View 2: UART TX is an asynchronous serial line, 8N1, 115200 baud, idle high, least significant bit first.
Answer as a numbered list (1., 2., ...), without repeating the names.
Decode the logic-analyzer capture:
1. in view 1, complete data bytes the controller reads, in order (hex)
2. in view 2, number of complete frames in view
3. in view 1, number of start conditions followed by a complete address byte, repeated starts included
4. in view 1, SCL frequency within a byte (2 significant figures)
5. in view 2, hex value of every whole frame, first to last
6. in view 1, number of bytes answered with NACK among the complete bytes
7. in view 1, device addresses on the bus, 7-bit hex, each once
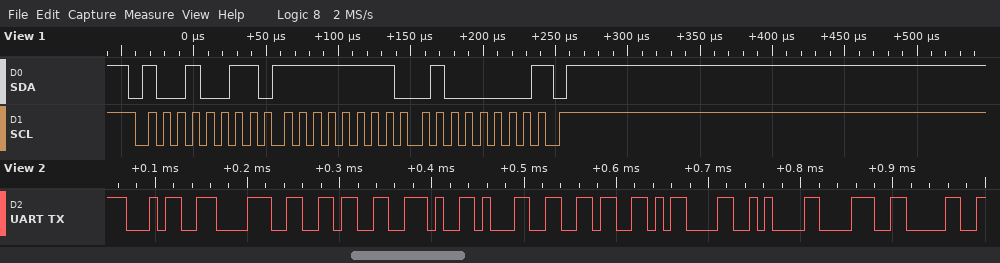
1. FF 40
2. 10
3. 1
4. 100 kHz
5. 34 38 36 2E 31 36 0D 0A 38 30
6. 1
7. 0x49
